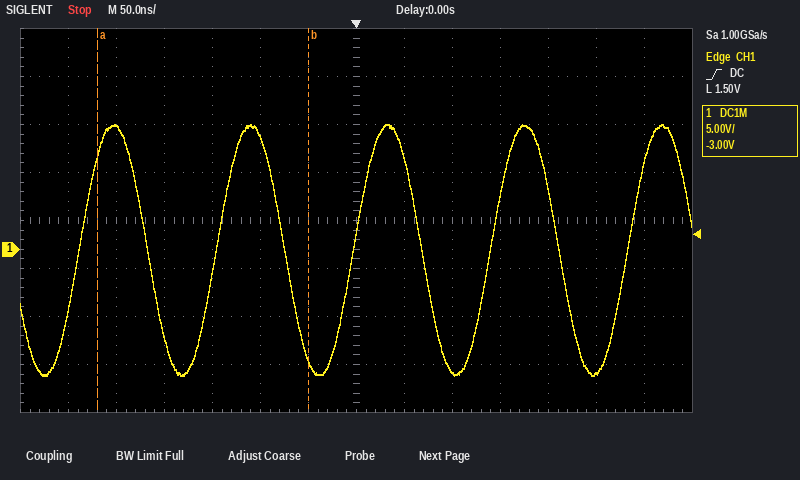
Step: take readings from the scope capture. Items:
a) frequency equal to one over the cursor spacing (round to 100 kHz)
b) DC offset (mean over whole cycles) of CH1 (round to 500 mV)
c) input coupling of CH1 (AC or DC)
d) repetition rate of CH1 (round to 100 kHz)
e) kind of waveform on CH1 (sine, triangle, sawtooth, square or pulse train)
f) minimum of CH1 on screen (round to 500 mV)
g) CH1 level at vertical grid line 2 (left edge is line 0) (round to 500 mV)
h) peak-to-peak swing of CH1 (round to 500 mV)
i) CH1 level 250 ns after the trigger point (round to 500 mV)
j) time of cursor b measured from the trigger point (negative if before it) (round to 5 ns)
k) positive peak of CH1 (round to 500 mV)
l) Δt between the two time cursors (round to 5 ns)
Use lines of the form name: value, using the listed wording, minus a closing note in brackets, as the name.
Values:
frequency equal to one over the cursor spacing: 4.5 MHz
DC offset (mean over whole cycles) of CH1: 0.0 V
input coupling of CH1: DC
repetition rate of CH1: 7.0 MHz
kind of waveform on CH1: sine
minimum of CH1 on screen: -13.0 V
CH1 level at vertical grid line 2 (left edge is line 0): 13.0 V
peak-to-peak swing of CH1: 26.0 V
CH1 level 250 ns after the trigger point: -13.0 V
time of cursor b measured from the trigger point (negative if before it): -50 ns
positive peak of CH1: 13.0 V
Δt between the two time cursors: 220 ns
